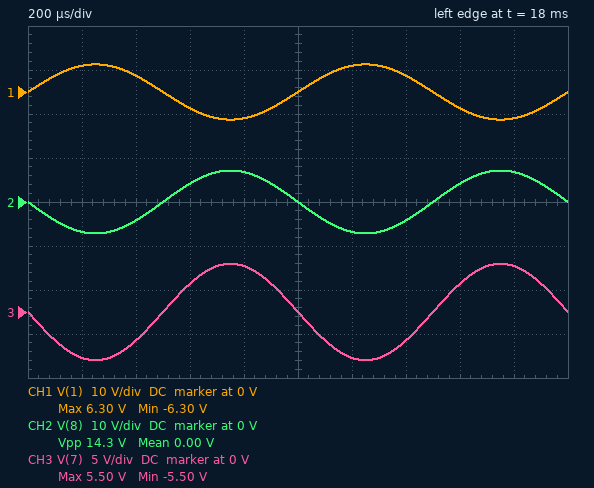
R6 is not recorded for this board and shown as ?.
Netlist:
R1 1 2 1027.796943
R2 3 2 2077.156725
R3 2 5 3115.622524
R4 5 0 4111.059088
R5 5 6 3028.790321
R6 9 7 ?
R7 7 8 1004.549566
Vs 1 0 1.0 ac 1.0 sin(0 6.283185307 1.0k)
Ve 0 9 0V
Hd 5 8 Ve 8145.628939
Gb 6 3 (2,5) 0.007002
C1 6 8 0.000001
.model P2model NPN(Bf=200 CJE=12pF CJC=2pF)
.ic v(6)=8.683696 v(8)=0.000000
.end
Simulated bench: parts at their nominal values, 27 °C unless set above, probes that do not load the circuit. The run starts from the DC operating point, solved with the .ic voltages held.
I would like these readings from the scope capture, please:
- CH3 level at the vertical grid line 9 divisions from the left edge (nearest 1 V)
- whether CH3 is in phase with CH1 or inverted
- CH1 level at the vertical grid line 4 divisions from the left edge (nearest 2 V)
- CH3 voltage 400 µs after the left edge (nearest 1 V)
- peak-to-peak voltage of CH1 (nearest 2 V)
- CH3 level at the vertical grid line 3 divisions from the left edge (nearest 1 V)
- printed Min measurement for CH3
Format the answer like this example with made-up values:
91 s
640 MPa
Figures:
5 V
inverted
-6 V
-3 V
12 V
3 V
-5.50 V
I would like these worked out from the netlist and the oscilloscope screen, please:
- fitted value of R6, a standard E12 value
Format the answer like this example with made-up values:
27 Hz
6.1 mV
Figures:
3.3 kΩ
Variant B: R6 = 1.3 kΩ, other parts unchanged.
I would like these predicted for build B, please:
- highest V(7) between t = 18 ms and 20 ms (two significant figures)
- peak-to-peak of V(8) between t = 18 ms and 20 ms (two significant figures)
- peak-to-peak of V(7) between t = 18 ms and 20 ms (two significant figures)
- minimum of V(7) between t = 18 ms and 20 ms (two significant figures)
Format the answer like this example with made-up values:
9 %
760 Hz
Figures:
1.3 V
4.7 V
2.6 V
-1.3 V
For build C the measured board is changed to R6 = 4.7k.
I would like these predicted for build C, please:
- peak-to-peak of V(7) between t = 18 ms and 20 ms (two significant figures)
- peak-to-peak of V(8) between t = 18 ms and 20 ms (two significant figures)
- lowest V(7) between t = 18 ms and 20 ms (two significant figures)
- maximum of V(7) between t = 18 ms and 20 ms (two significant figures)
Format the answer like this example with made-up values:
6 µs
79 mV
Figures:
28 V
34 V
-14 V
14 V
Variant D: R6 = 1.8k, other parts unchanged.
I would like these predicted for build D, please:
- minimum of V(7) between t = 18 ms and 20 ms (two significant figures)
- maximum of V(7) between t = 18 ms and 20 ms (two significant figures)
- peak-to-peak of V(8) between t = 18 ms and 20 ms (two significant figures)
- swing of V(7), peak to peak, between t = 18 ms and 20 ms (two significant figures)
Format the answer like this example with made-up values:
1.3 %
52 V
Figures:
-2.0 V
2.0 V
6.3 V
4.0 V
